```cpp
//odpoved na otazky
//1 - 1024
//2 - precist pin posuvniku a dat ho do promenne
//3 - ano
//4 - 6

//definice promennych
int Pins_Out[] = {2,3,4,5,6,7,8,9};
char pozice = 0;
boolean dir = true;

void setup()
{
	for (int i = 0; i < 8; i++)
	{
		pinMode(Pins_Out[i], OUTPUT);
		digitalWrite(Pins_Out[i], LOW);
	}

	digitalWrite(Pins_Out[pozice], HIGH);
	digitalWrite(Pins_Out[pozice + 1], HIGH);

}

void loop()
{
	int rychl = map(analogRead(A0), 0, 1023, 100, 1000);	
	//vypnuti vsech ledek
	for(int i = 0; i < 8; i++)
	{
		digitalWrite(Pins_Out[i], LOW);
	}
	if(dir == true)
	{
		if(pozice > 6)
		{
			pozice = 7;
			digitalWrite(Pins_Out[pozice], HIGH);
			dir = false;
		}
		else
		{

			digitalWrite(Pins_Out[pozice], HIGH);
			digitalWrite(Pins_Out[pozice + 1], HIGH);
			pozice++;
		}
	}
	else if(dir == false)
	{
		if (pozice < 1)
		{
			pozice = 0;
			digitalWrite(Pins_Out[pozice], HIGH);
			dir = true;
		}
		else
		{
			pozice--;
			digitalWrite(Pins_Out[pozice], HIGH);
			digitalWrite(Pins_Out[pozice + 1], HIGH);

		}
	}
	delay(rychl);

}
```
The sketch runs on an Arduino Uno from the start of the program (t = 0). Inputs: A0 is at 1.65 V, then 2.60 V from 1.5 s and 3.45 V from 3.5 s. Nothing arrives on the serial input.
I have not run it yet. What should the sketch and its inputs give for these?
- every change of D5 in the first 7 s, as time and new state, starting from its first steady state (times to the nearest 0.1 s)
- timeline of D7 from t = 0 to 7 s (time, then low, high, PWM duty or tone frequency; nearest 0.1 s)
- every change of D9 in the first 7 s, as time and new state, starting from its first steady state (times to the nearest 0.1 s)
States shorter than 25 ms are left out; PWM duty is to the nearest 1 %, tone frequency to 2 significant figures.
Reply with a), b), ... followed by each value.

a) 0 s low; 0.8 s high; 1.6 s low; 6 s high
b) 0 s low; 1.6 s high; 2.7 s low; 4.6 s high; 6 s low
c) 0 s low; 2.7 s high; 4.6 s low
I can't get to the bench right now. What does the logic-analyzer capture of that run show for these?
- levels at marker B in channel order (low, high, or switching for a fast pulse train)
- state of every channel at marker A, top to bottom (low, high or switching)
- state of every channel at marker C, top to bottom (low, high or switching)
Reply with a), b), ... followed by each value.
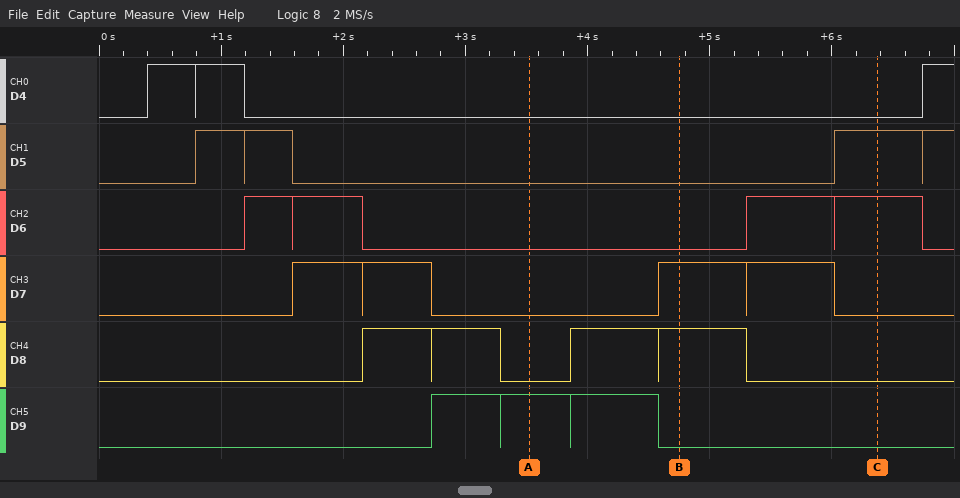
a) D4 low, D5 low, D6 low, D7 high, D8 high, D9 low
b) D4 low, D5 low, D6 low, D7 low, D8 low, D9 high
c) D4 low, D5 high, D6 high, D7 low, D8 low, D9 low
